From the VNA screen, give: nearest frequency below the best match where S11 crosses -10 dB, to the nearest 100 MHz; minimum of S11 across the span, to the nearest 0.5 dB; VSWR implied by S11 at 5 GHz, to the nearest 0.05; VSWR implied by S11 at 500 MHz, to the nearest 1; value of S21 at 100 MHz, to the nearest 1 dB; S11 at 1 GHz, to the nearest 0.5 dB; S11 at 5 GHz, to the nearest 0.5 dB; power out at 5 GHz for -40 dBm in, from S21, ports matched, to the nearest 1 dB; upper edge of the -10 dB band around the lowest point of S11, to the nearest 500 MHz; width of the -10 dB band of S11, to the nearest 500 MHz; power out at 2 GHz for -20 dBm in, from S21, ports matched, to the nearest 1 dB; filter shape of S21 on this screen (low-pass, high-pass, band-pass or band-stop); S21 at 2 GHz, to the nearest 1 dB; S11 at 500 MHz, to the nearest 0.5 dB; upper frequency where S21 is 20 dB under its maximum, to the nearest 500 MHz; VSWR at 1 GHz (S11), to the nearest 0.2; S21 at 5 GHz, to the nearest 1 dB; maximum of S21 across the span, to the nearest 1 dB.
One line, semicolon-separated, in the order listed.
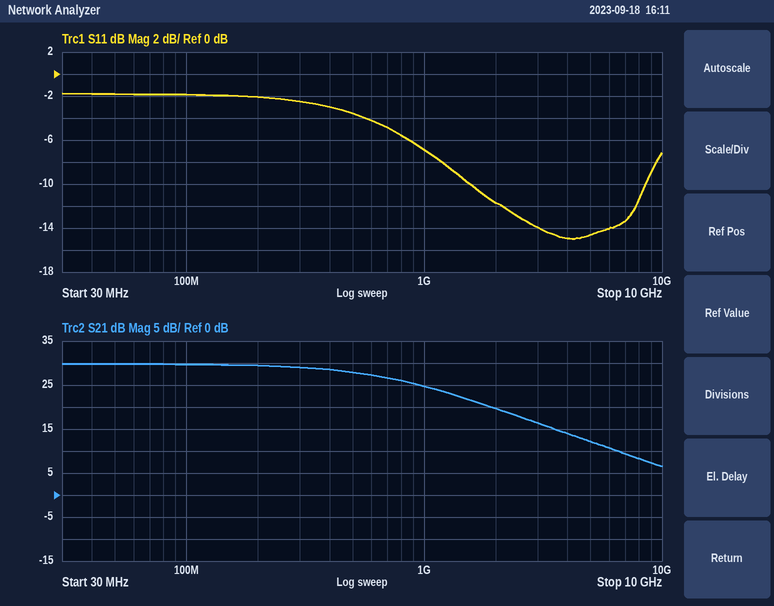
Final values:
1.6 GHz; -15.0 dB; 1.45; 5; 30 dB; -7.0 dB; -14.5 dB; -28 dBm; 8.5 GHz; 7.0 GHz; 0 dBm; low-pass; 20 dB; -3.5 dB; 6.5 GHz; 2.6; 12 dB; 30 dB
